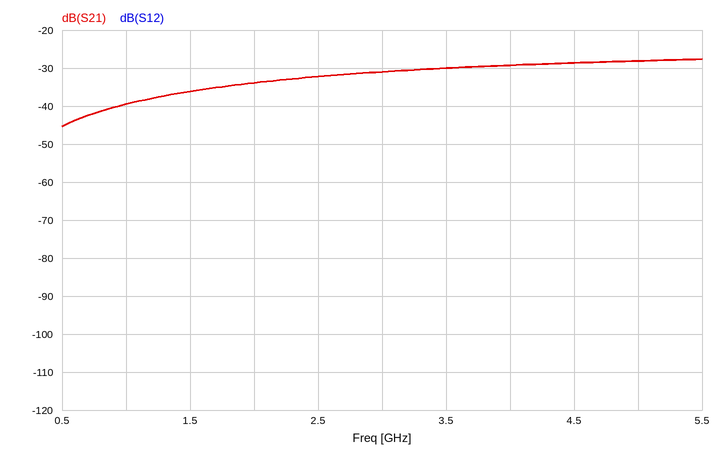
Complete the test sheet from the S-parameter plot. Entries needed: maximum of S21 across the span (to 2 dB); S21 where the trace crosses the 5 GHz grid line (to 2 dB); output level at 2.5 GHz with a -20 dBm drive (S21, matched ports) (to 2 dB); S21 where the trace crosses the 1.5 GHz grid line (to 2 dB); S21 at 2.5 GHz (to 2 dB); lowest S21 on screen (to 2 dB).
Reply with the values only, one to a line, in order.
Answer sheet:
-28 dB
-28 dB
-52 dBm
-36 dB
-32 dB
-46 dB
